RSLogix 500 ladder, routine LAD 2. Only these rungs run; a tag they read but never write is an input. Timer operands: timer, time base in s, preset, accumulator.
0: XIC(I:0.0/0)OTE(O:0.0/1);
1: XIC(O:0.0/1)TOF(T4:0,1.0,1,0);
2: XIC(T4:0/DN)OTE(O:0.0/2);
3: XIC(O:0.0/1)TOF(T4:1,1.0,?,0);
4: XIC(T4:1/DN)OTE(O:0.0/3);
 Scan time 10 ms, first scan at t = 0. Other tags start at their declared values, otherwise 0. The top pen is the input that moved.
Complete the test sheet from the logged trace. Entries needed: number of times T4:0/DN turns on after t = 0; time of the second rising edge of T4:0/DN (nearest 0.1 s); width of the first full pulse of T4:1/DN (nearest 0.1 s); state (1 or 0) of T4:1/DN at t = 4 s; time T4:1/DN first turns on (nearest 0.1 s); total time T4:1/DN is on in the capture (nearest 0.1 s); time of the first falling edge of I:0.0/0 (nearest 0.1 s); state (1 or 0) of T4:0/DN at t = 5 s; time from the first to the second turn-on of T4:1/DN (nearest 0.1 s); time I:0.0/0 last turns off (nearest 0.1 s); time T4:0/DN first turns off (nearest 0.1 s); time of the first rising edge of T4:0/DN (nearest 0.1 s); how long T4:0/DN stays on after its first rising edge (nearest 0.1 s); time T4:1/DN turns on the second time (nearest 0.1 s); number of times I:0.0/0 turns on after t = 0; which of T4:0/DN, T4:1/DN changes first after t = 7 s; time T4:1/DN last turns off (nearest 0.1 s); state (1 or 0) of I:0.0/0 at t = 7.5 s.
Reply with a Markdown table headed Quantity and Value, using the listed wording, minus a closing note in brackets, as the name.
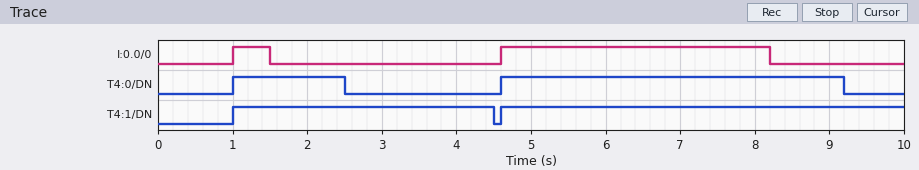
| Quantity | Value |
|---|---|
| number of times T4:0/DN turns on after t = 0 | 2 |
| time of the second rising edge of T4:0/DN | 4.6 s |
| width of the first full pulse of T4:1/DN | 3.5 s |
| state (1 or 0) of T4:1/DN at t = 4 s | 1 |
| time T4:1/DN first turns on | 1.0 s |
| total time T4:1/DN is on in the capture | 8.9 s |
| time of the first falling edge of I:0.0/0 | 1.5 s |
| state (1 or 0) of T4:0/DN at t = 5 s | 1 |
| time from the first to the second turn-on of T4:1/DN | 3.6 s |
| time I:0.0/0 last turns off | 8.2 s |
| time T4:0/DN first turns off | 2.5 s |
| time of the first rising edge of T4:0/DN | 1.0 s |
| how long T4:0/DN stays on after its first rising edge | 1.5 s |
| time T4:1/DN turns on the second time | 4.6 s |
| number of times I:0.0/0 turns on after t = 0 | 2 |
| which of T4:0/DN, T4:1/DN changes first after t = 7 s | T4:0/DN |
| time T4:1/DN last turns off | 4.5 s |
| state (1 or 0) of I:0.0/0 at t = 7.5 s | 1 |
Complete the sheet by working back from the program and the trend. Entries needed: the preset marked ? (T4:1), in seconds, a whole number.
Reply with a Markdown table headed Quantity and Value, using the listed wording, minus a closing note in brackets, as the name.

| Quantity | Value |
|---|---|
| the preset marked ? (T4:1), in seconds, a whole number | 3 s |
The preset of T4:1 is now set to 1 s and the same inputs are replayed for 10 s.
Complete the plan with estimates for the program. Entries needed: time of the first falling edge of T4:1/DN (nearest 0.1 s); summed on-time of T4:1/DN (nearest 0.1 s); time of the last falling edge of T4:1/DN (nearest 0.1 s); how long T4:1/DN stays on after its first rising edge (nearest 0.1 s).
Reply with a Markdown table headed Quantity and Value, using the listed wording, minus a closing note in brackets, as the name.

| Quantity | Value |
|---|---|
| time of the first falling edge of T4:1/DN | 2.5 s |
| summed on-time of T4:1/DN | 6.1 s |
| time of the last falling edge of T4:1/DN | 9.2 s |
| how long T4:1/DN stays on after its first rising edge | 1.5 s |
